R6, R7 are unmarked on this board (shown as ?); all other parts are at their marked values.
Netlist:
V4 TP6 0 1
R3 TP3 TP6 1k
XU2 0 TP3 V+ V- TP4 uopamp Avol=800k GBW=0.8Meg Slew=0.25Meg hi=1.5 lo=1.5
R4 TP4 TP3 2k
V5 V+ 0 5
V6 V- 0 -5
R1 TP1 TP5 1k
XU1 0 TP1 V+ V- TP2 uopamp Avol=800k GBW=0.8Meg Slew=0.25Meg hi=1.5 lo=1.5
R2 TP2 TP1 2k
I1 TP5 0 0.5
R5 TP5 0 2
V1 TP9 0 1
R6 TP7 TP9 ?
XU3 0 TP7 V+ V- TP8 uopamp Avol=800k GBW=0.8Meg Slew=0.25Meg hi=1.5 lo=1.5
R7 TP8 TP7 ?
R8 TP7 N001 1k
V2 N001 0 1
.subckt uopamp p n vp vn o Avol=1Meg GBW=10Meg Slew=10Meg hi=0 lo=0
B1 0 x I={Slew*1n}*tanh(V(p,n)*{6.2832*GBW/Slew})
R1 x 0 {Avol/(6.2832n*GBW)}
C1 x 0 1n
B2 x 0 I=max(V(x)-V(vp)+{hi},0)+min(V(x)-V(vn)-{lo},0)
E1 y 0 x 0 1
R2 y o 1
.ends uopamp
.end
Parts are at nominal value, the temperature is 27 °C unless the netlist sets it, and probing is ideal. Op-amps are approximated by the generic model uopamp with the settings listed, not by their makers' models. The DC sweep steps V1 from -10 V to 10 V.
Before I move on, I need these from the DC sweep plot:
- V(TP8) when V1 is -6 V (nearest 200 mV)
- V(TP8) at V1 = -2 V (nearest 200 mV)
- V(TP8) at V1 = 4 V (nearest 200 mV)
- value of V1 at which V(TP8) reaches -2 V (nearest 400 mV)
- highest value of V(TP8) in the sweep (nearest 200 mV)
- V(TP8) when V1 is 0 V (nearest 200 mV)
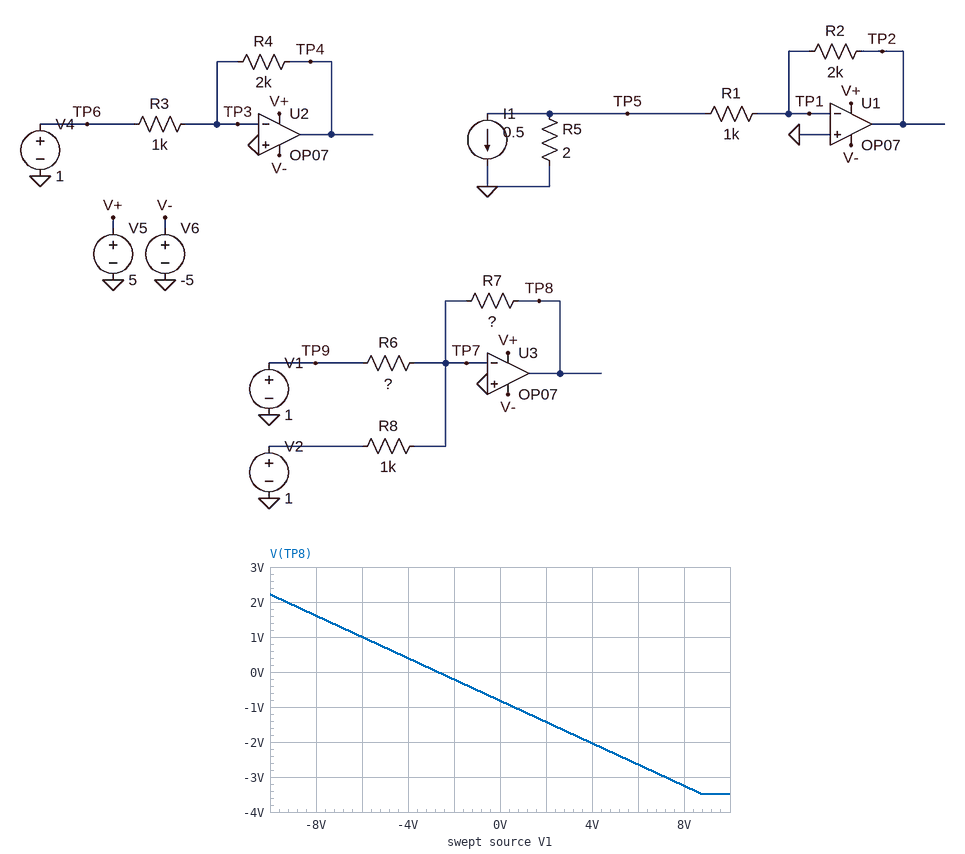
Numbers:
1.0 V
-200 mV
-2.0 V
4.0 V
2.2 V
-800 mV
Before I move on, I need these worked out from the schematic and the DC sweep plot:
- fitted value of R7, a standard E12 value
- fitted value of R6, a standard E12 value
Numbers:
820 Ω
2.7 kΩ
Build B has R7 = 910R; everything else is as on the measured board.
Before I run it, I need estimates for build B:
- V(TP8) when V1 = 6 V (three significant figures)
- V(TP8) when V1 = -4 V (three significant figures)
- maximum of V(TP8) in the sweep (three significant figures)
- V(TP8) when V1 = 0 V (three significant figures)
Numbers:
-2.93 V
438 mV
2.46 V
-910 mV
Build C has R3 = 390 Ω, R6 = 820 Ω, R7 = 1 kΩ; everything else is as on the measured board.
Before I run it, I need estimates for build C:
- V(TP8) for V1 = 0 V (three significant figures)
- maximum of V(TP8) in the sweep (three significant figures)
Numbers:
-1.00 V
3.50 V
